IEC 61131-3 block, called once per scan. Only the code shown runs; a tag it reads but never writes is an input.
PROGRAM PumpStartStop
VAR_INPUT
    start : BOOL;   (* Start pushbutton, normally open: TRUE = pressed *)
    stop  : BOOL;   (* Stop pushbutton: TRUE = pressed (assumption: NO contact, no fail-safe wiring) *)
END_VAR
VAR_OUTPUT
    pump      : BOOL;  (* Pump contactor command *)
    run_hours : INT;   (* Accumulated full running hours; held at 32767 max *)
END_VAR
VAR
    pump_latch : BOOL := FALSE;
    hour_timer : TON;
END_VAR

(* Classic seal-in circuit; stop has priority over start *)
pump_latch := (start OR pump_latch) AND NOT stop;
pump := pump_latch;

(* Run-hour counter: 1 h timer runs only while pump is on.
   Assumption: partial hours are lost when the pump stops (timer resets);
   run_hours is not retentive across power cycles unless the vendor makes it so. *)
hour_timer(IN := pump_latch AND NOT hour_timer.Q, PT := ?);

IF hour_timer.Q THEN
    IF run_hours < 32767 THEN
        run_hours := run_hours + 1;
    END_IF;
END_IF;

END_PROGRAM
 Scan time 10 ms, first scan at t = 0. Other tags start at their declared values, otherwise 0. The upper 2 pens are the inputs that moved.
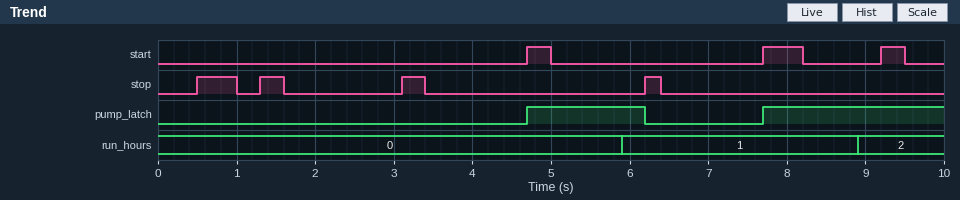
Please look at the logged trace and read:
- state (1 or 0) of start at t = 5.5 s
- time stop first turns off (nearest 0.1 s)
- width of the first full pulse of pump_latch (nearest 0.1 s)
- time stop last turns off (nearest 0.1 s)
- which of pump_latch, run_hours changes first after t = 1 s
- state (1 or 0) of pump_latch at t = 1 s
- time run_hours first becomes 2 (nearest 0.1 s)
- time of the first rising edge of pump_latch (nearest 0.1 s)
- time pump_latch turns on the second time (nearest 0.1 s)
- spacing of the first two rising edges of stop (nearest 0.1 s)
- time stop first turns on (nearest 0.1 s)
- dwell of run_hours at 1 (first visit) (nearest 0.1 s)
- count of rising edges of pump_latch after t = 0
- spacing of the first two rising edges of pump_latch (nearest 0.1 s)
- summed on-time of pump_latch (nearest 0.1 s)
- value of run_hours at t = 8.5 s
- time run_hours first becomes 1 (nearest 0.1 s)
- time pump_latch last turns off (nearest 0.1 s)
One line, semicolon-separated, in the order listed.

0; 1.0 s; 1.5 s; 6.4 s; pump_latch; 0; 8.9 s; 4.7 s; 7.7 s; 0.8 s; 0.5 s; 3.0 s; 2; 3.0 s; 3.8 s; 1; 5.9 s; 6.2 s
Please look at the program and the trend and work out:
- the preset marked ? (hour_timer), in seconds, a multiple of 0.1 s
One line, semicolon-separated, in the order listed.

1.2 s
